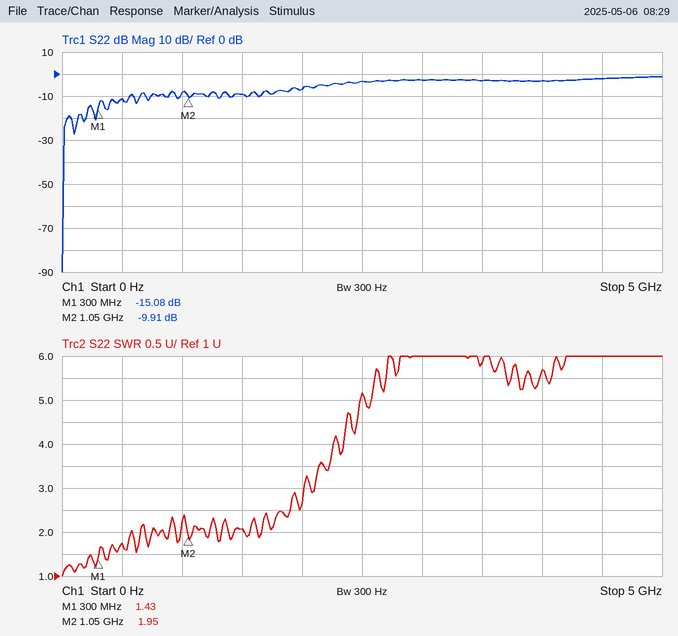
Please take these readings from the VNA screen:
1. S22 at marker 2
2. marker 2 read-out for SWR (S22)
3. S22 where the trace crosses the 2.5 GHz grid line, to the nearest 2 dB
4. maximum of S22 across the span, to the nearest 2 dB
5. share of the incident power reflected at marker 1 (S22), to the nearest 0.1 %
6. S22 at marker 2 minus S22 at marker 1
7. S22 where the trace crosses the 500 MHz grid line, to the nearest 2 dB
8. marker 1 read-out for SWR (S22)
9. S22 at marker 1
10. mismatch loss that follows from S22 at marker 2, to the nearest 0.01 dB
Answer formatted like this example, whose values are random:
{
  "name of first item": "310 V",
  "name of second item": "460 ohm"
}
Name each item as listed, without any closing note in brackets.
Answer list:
{
  "S22 at marker 2": "-9.91 dB",
  "marker 2 read-out for SWR": "1.95",
  "S22 where the trace crosses the 2.5 GHz grid line, to the nearest 2 dB": "-4 dB",
  "maximum of S22 across the span, to the nearest 2 dB": "-2 dB",
  "share of the incident power reflected at marker 1 (S22), to the nearest 0.1 %": "3.1 %",
  "S22 at marker 2 minus S22 at marker 1": "5.17 dB",
  "S22 where the trace crosses the 500 MHz grid line, to the nearest 2 dB": "-12 dB",
  "marker 1 read-out for SWR": "1.43",
  "S22 at marker 1": "-15.08 dB",
  "mismatch loss that follows from S22 at marker 2, to the nearest 0.01 dB": "0.47 dB"
}
